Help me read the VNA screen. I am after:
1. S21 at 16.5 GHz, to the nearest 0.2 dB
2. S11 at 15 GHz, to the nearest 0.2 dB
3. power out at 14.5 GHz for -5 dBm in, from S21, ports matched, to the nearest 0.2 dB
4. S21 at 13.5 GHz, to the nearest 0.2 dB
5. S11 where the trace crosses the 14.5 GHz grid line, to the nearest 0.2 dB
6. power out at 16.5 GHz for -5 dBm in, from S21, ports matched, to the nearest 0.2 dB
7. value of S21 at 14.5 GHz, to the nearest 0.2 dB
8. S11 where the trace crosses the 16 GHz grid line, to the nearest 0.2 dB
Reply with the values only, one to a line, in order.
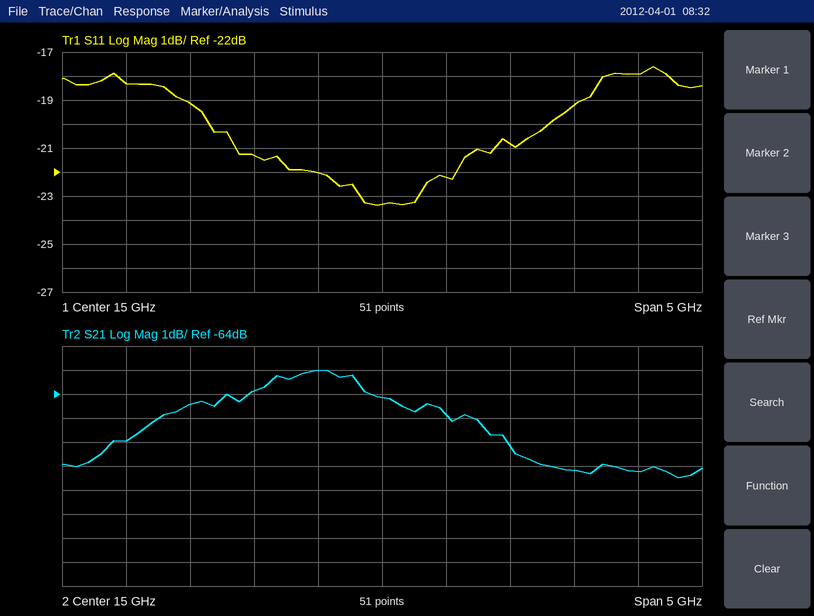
-67.2 dB
-23.4 dB
-68.0 dBm
-64.4 dB
-22.0 dB
-72.2 dBm
-63.0 dB
-20.8 dB
